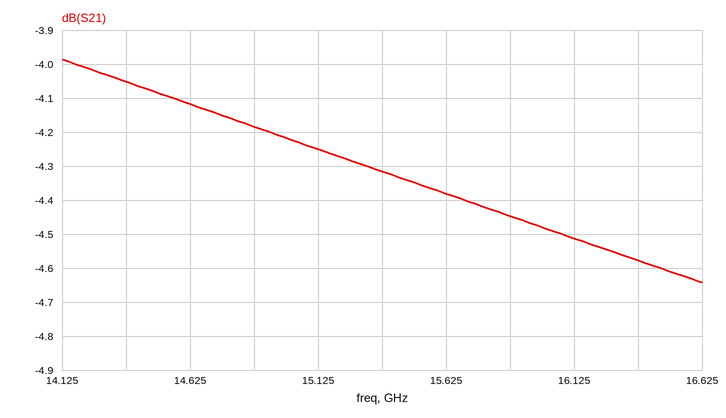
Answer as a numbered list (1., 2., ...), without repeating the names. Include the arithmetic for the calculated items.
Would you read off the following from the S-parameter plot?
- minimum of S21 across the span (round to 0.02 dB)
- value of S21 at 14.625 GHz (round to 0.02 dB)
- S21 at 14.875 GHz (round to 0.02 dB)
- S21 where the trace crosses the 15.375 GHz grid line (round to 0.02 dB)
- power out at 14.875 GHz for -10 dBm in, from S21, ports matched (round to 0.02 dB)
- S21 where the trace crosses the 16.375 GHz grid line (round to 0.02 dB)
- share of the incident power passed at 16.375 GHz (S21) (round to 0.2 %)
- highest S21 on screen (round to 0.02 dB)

1. -4.64 dB
2. -4.12 dB
3. -4.18 dB
4. -4.32 dB
5. -10 dBm + (-4.18 dB) = -14.18 dBm
6. -4.58 dB
7. 10^(-4.58/10) ≈ 34.8 %
8. -3.98 dB
